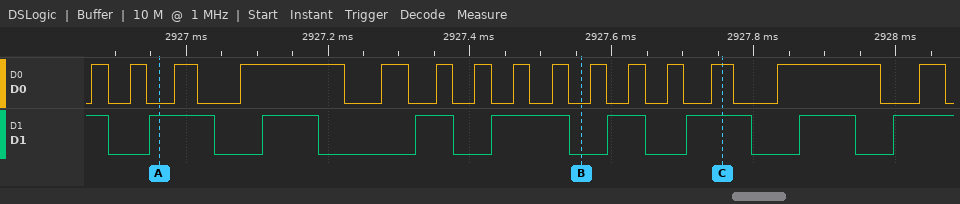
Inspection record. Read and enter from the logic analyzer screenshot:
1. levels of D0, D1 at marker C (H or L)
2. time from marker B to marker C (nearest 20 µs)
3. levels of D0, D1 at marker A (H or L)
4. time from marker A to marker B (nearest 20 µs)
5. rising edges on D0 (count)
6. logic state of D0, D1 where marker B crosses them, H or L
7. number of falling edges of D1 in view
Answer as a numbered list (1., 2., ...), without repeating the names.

1. D0=H, D1=H
2. 200 µs
3. D0=L, D1=H
4. 600 µs
5. 15
6. D0=L, D1=L
7. 8
